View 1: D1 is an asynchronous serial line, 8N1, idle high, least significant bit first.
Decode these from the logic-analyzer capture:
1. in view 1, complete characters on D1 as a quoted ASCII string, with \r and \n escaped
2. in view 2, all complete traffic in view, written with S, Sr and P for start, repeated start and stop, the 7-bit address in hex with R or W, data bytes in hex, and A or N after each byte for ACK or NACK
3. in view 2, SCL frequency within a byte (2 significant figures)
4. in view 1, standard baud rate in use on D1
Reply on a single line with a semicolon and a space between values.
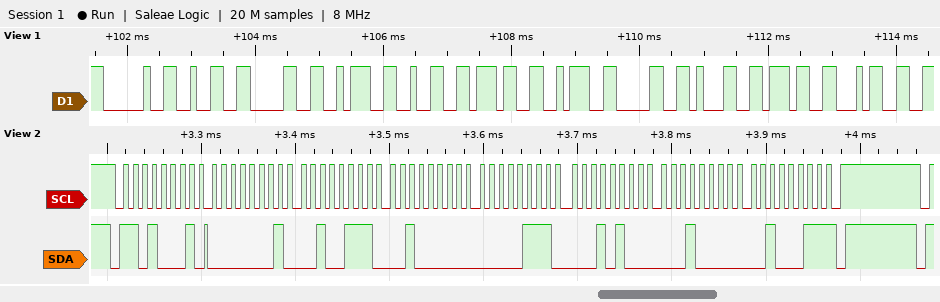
" 20:27:0174"; S 68R A 01 A 27 A 20 A 07 A 14 A 10 A 23 N P; 100 kHz; 9600 baud
